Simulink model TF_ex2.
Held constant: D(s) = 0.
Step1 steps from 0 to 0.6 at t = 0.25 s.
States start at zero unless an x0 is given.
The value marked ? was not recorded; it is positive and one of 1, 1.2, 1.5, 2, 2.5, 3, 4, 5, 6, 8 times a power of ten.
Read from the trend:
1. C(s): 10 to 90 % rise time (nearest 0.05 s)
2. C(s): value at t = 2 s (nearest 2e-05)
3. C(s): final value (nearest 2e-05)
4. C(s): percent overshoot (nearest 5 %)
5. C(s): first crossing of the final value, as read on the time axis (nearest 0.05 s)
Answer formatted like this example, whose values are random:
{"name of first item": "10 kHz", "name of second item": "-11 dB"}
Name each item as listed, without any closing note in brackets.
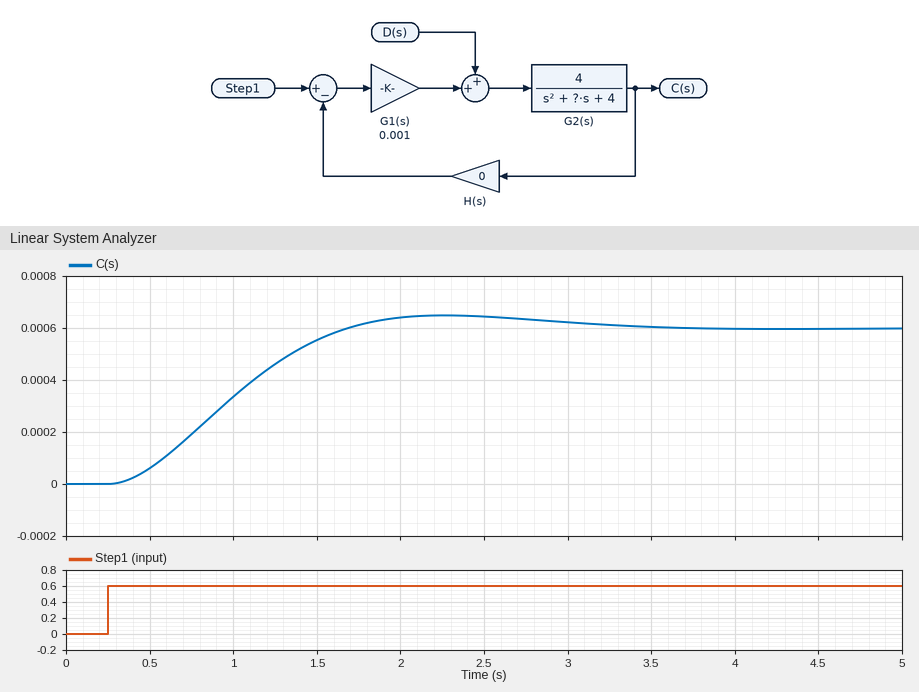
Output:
{"C(s): 10 to 90 % rise time": "0.95 s", "C(s): value at t = 2 s": "0.00064", "C(s): final value": "0.00060", "C(s): percent overshoot": "10 %", "C(s): first crossing of the final value, as read on the time axis": "1.70 s"}
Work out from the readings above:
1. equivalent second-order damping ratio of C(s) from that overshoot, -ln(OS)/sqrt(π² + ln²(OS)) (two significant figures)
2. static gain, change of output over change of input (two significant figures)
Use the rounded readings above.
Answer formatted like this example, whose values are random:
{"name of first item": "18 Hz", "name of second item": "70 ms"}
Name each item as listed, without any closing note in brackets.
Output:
{"equivalent second-order damping ratio of C(s) from that overshoot, -ln(OS)/sqrt(π² + ln²(OS))": "0.59", "static gain, change of output over change of input": "0.0010"}
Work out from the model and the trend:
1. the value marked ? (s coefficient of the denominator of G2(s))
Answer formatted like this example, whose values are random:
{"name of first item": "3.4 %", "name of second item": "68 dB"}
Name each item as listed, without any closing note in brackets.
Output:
{"the value marked ? (s coefficient of the denominator of G2(s))": "2.5"}
